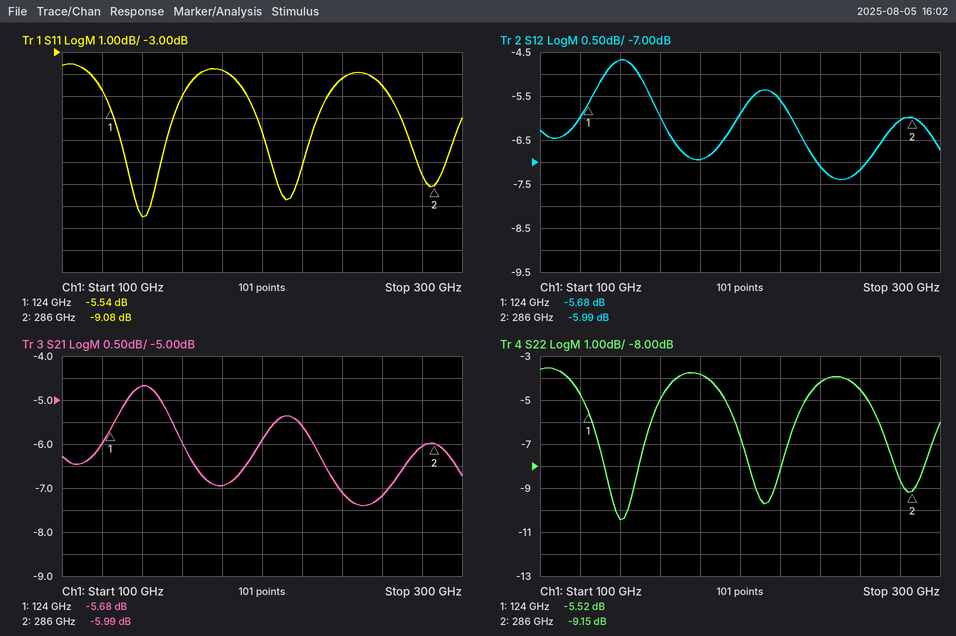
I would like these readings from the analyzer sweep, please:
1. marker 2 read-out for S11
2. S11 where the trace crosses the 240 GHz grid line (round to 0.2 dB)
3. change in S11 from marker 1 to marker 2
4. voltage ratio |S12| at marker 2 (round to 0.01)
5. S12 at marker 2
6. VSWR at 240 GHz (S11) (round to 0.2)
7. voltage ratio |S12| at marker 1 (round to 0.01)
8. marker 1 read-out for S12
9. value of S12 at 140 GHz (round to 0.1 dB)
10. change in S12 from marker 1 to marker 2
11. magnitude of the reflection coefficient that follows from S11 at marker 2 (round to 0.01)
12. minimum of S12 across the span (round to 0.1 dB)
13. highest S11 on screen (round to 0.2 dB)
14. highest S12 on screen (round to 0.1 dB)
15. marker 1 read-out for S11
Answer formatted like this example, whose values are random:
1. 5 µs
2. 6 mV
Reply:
1. -9.08 dB
2. -4.2 dB
3. -3.54 dB
4. 0.50
5. -5.99 dB
6. 4.2
7. 0.52
8. -5.68 dB
9. -4.7 dB
10. -0.31 dB
11. 0.35
12. -7.4 dB
13. -3.6 dB
14. -4.7 dB
15. -5.54 dB
